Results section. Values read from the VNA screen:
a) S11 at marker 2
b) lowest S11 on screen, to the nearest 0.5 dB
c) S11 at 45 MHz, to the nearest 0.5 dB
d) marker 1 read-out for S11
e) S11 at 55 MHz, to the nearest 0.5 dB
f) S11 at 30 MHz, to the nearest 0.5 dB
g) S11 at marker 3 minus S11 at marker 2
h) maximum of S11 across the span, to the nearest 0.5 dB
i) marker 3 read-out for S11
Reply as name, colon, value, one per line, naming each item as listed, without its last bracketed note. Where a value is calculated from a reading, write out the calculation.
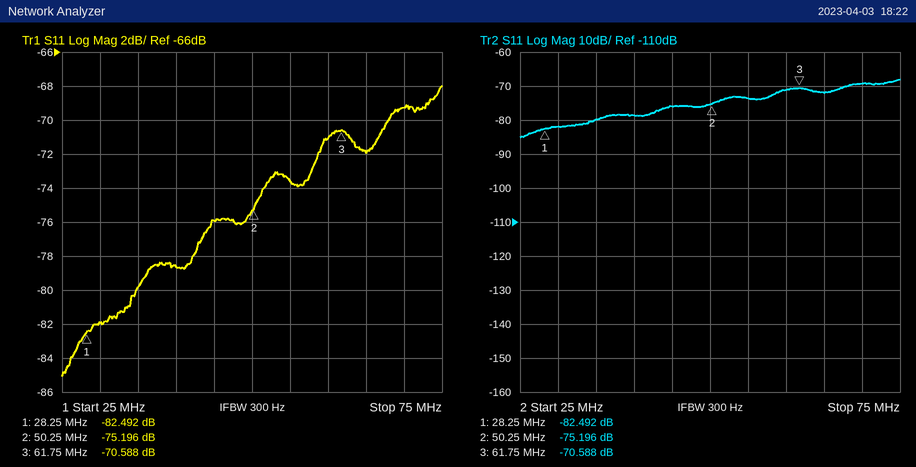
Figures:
S11 at marker 2: -75.196 dB
lowest S11 on screen, to the nearest 0.5 dB: -85.0 dB
S11 at 45 MHz, to the nearest 0.5 dB: -76.0 dB
marker 1 read-out for S11: -82.492 dB
S11 at 55 MHz, to the nearest 0.5 dB: -73.5 dB
S11 at 30 MHz, to the nearest 0.5 dB: -82.0 dB
S11 at marker 3 minus S11 at marker 2: -70.588 − (-75.196) = 4.608 dB
maximum of S11 across the span, to the nearest 0.5 dB: -68.0 dB
marker 3 read-out for S11: -70.588 dB
